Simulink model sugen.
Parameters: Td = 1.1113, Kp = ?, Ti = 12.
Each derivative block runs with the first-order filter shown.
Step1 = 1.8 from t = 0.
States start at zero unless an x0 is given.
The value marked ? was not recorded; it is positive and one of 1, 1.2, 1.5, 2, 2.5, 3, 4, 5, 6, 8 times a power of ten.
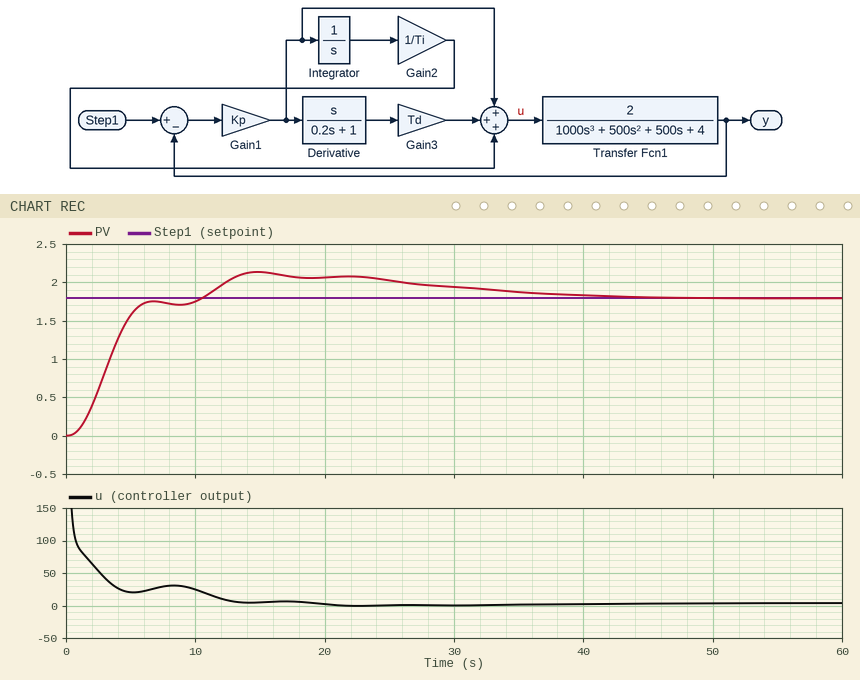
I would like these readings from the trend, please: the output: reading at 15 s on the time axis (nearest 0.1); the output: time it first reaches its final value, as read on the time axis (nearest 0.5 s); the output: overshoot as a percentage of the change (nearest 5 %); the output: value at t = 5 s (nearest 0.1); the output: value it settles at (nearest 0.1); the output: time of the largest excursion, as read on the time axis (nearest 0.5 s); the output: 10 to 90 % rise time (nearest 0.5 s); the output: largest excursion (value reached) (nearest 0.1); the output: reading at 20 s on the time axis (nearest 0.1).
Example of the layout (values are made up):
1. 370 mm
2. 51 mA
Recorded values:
1. 2.1
2. 10.5 s
3. 20 %
4. 1.6
5. 1.8
6. 15.0 s
7. 4.0 s
8. 2.1
9. 2.1
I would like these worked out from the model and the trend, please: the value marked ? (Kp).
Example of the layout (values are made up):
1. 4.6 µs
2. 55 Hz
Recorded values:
1. 50
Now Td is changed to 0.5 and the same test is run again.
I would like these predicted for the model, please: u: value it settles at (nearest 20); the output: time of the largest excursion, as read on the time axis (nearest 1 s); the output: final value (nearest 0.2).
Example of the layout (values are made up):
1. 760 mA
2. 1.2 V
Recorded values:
1. 0
2. 16 s
3. 1.8
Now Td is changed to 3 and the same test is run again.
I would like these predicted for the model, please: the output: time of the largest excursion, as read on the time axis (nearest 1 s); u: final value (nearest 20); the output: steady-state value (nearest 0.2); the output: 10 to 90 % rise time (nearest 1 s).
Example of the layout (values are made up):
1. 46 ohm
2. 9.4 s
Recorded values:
1. 19 s
2. 0
3. 1.8
4. 3 s
